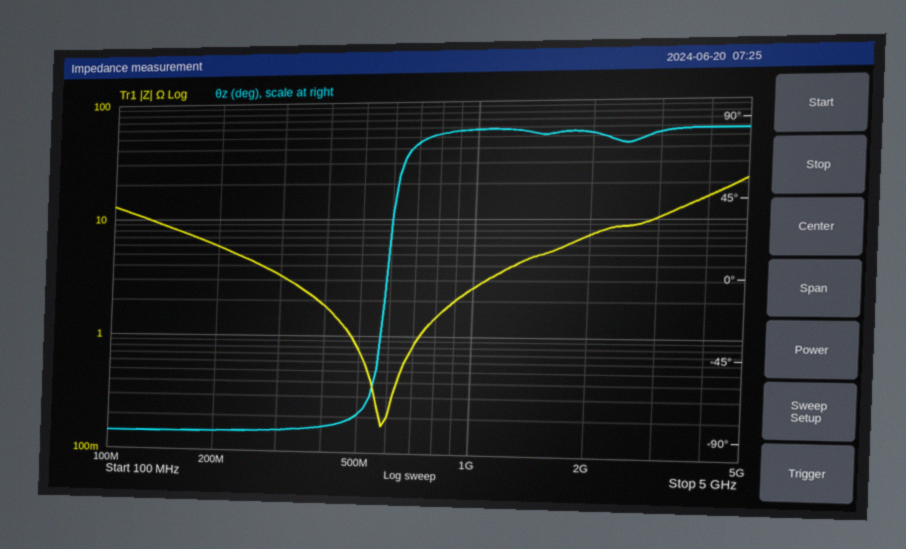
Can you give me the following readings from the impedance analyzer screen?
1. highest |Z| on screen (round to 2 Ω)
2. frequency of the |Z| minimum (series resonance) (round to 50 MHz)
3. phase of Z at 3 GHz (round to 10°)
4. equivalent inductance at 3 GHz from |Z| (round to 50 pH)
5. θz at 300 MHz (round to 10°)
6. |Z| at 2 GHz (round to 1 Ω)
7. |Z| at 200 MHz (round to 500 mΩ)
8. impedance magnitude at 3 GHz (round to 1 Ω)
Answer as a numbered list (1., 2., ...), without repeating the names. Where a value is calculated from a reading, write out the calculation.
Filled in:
1. 22 Ω
2. 600 MHz
3. 80°
4. L = 10 Ω/(2π × 3 GHz) ≈ 531 pH, so 550 pH to the nearest 50 pH
5. -90°
6. 7 Ω
7. 6.0 Ω
8. 10 Ω
